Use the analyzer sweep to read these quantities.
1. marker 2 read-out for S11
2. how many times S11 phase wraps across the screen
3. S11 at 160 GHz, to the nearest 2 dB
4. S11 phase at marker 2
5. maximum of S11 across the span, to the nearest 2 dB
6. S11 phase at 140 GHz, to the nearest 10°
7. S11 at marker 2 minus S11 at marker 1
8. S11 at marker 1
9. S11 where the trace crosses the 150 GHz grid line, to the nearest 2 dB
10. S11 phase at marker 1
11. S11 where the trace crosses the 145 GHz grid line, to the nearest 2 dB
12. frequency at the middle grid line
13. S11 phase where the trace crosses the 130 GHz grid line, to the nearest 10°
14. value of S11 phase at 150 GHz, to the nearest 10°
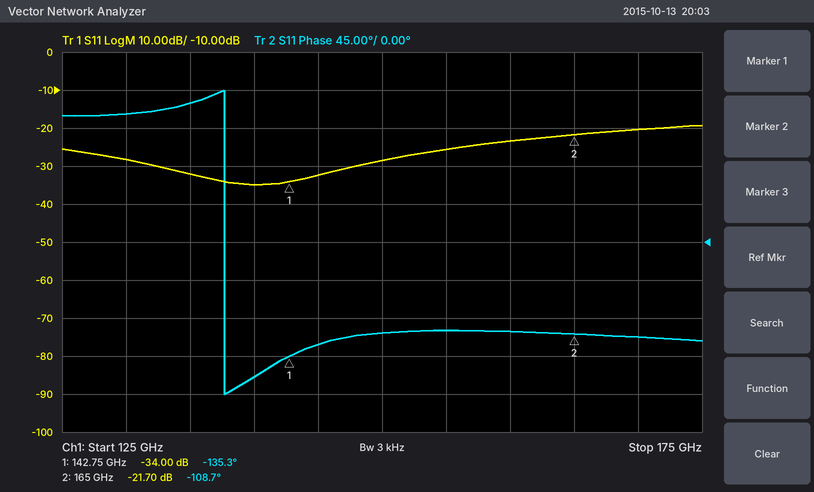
-21.70 dB
1
-24 dB
-108.7°
-20 dB
-160°
12.30 dB
-34.00 dB
-28 dB
-135.3°
-32 dB
150 GHz
150°
-110°
